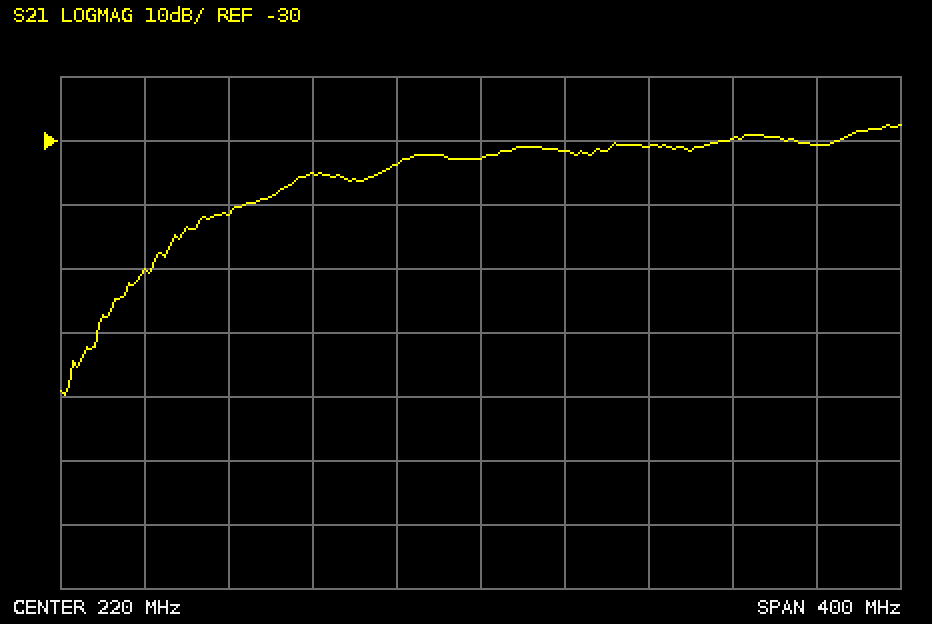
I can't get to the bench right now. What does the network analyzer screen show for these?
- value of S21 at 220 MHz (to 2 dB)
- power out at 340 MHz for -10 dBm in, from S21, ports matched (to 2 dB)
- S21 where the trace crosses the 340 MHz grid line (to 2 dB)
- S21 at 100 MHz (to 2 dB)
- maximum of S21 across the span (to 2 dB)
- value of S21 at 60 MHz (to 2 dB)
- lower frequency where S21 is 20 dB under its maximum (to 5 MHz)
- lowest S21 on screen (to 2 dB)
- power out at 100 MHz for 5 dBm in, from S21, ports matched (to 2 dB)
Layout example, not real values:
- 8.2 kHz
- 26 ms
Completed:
- -32 dB
- -40 dBm
- -30 dB
- -42 dB
- -28 dB
- -50 dB
- 70 MHz
- -70 dB
- -36 dBm
